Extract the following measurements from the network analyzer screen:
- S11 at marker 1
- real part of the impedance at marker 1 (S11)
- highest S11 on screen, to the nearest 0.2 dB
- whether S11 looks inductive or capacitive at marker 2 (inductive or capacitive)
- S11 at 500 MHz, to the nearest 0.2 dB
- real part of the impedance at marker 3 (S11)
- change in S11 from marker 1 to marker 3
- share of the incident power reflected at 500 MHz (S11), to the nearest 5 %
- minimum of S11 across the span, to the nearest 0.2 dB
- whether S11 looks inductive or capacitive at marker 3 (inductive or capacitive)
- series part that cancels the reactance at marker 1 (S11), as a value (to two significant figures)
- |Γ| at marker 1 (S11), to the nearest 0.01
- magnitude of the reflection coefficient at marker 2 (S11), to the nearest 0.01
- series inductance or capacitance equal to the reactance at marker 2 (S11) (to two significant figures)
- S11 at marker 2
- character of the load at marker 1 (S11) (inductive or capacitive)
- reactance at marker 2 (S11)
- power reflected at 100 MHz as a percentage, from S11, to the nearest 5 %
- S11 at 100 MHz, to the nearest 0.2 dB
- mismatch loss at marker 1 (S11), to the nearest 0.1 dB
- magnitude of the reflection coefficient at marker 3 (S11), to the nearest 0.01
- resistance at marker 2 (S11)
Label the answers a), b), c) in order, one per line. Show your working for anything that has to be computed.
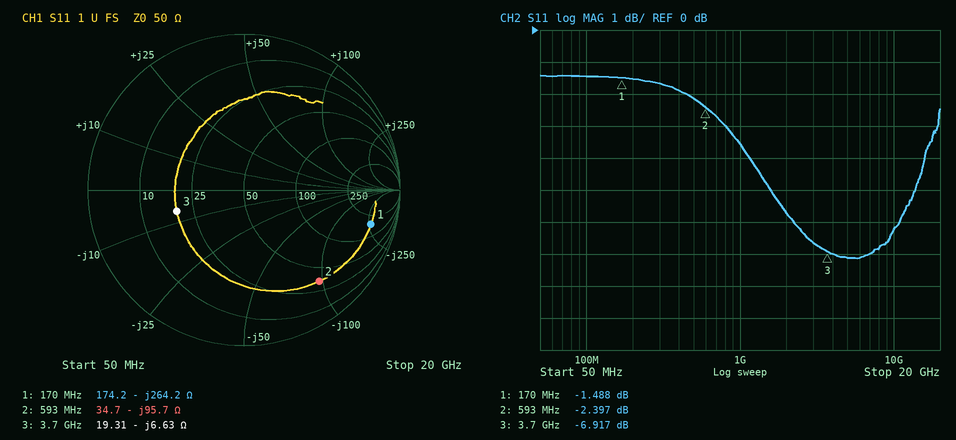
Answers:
a) -1.488 dB
b) 174.2 Ω
c) -1.4 dB
d) capacitive
e) -2.2 dB
f) 19.31 Ω
g) -6.917 − (-1.488) = -5.429 dB
h) 10^(-2.2/10) ≈ 60 %
i) -7.2 dB
j) capacitive
k) L = 264.2 Ω/(2π × 170 MHz) ≈ 247 nH, so 250 nH to two significant figures
l) 0.84
m) 0.76
n) C = 1/(2π × 593 MHz × 95.7 Ω) ≈ 2.8 pF
o) -2.397 dB
p) capacitive
q) -95.7 Ω
r) 10^(-1.4/10) ≈ 72.4 %, so 70 % to the nearest 5 %
s) -1.4 dB
t) −10 log10(1 − 10^(-1.488/10)) ≈ 5.4 dB
u) 10^(-6.917/20) ≈ 0.45
v) 34.7 Ω
